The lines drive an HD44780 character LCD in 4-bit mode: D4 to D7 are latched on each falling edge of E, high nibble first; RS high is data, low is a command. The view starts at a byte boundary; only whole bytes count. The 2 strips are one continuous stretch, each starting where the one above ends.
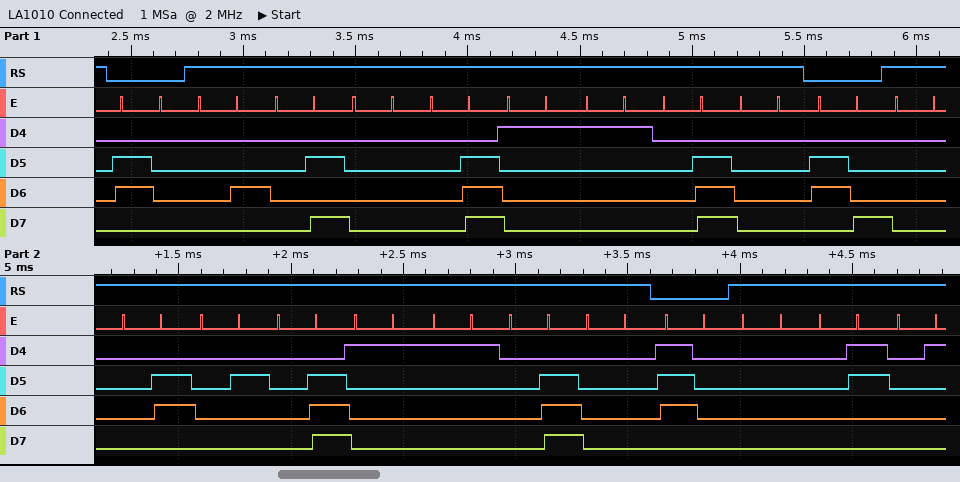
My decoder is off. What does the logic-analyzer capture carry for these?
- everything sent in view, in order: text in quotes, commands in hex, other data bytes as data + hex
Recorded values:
0x60 data 04 0A 00 0E 11 11 0E 00 0x68 data 00 06 02 0E 11 11 0E 00 0x70 data 00 03 01
